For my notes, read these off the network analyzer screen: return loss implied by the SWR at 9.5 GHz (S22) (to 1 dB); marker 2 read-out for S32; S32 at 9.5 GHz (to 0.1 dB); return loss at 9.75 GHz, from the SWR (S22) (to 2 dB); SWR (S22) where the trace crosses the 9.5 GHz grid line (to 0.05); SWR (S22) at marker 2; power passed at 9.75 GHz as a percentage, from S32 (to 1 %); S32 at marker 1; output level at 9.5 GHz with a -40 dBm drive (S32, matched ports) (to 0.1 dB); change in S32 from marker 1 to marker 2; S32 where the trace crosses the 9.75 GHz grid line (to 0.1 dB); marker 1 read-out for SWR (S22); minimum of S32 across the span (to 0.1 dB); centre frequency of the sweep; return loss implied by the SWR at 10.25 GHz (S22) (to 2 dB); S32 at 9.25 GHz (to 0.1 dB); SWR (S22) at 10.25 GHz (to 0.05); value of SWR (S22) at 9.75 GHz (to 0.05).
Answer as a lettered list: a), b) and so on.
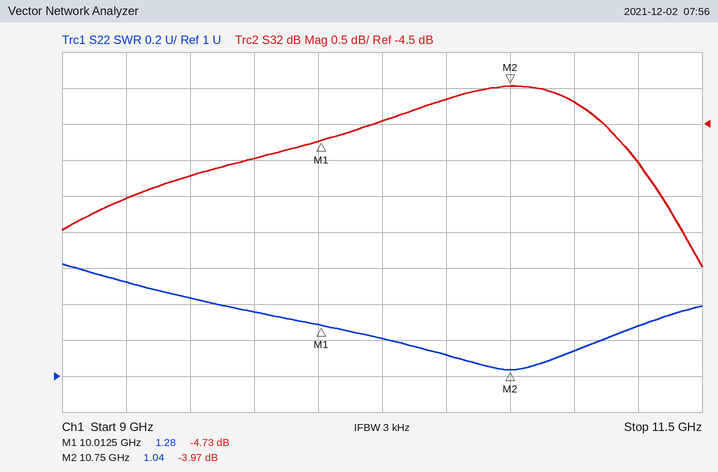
a) 15 dB
b) -3.97 dB
c) -5.2 dB
d) 16 dB
e) 1.45
f) 1.04
g) 32 %
h) -4.73 dB
i) -45.2 dBm
j) 0.76 dB
k) -5.0 dB
l) 1.28
m) -6.5 dB
n) 10.25 GHz
o) 20 dB
p) -5.5 dB
q) 1.20
r) 1.35
